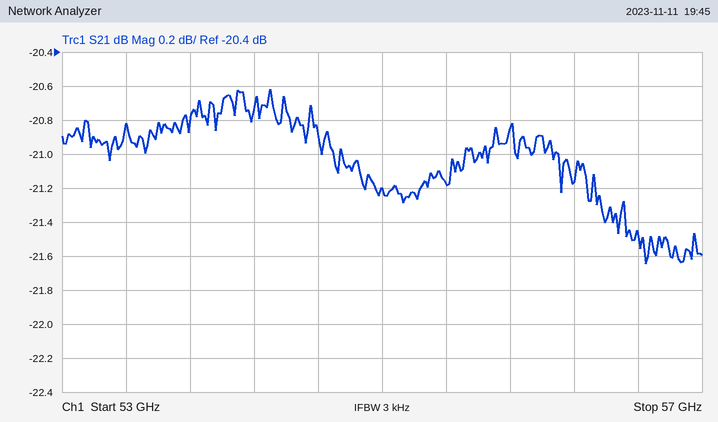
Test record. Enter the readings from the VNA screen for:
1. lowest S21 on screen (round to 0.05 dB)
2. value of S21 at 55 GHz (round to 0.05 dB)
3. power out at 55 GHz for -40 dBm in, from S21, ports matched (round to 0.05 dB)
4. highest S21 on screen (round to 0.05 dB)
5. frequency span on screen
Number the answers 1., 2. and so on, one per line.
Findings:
1. -21.65 dB
2. -21.20 dB
3. -61.20 dBm
4. -20.60 dB
5. 4 GHz
